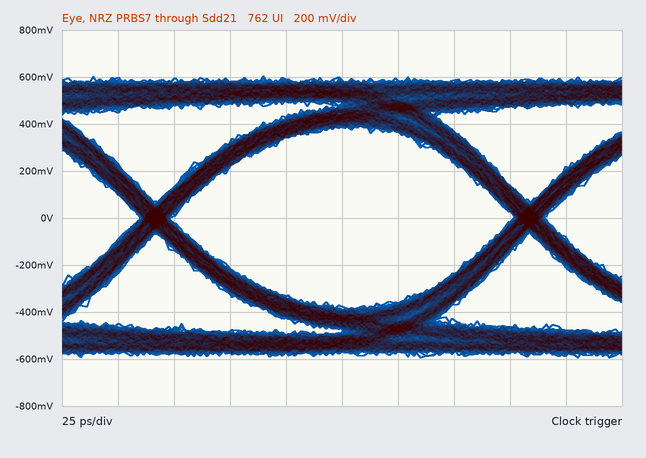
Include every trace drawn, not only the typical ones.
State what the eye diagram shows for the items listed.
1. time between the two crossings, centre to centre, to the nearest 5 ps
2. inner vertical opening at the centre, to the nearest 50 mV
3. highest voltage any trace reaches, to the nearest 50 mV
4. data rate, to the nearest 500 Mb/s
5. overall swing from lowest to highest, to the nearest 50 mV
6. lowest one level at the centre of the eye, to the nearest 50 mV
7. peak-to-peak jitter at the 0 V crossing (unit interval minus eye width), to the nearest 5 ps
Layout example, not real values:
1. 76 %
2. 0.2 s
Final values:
1. 165 ps
2. 750 mV
3. 600 mV
4. 6.0 Gb/s
5. 1.20 V
6. 400 mV
7. 15 ps
